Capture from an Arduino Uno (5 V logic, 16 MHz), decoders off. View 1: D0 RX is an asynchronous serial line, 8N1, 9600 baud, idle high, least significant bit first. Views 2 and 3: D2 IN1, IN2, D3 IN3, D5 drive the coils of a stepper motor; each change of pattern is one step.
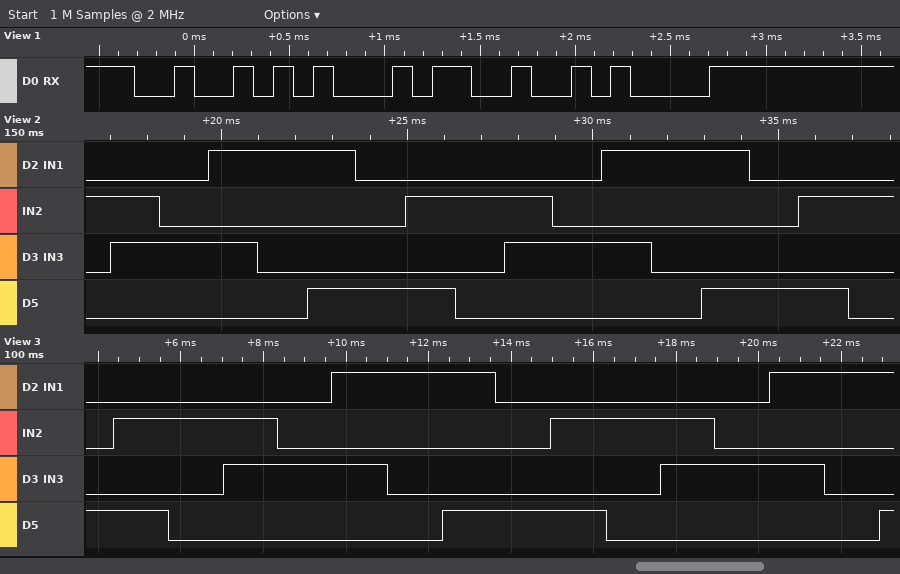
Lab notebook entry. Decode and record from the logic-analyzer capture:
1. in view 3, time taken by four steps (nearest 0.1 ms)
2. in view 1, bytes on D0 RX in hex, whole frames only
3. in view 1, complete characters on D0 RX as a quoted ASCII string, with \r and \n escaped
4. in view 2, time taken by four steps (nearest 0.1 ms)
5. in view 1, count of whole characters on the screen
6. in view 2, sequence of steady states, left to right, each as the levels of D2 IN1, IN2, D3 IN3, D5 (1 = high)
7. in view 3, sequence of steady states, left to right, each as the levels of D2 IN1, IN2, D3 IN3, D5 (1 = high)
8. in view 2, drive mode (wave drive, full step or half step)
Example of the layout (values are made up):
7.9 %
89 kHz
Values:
5.3 ms
52 34 0A
"R4\n"
5.3 ms
3
0100 0110 0010 1010 1000 1001 0001 0101 0100 0110 0010 1010 1000 1001 0001 0101 0100
0001 0101 0100 0110 0010 1010 1000 1001 0001 0101 0100 0110 0010 1010 1000 1001
half step
